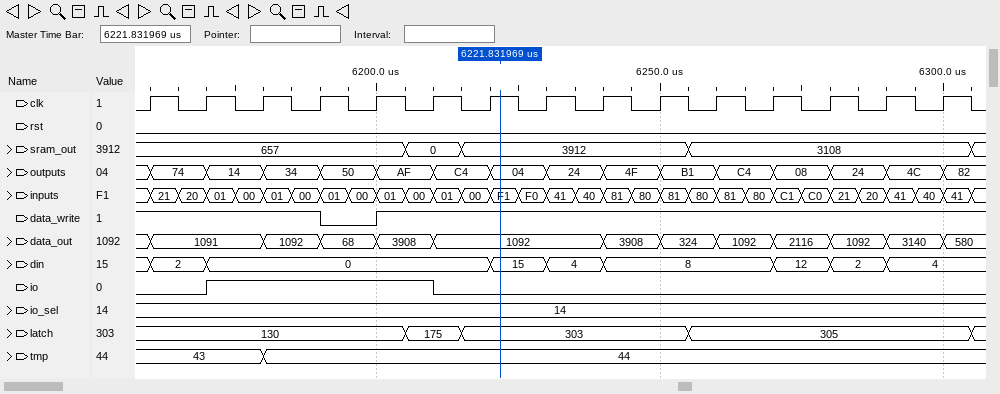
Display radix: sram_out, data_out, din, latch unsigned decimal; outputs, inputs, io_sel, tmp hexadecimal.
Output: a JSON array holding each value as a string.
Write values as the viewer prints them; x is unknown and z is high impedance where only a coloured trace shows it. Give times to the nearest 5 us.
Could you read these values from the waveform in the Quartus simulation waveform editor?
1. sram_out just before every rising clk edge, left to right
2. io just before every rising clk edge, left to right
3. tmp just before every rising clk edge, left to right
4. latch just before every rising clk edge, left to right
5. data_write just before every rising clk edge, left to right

["657, 657, 657, 657, 657, 0, 3912, 3912, 3912, 3912, 3108, 3108, 3108, 3108, 3108", "0 0 1 1 1 1 0 0 0 0 0 0 0 0 0", "43, 43, 43, 44, 44, 44, 44, 44, 44, 44, 44, 44, 44, 44, 44", "130, 130, 130, 130, 130, 175, 303, 303, 303, 303, 305, 305, 305, 305, 305", "1 1 1 1 0 1 1 1 1 1 1 1 1 1 1"]
